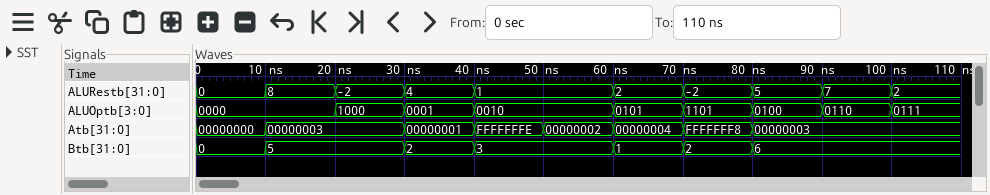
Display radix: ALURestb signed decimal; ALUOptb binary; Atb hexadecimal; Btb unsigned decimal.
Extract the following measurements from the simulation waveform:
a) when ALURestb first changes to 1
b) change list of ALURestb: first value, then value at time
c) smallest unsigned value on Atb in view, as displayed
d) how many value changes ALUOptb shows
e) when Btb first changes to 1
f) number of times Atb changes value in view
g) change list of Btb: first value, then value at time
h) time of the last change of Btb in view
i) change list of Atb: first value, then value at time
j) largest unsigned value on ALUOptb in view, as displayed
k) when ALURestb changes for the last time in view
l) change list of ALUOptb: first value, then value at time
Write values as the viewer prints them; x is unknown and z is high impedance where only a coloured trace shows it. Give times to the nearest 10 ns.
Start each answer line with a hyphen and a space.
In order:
- 40 ns
- 0, 8 at 10 ns, -2 at 20 ns, 4 at 30 ns, 1 at 40 ns, 2 at 60 ns, -2 at 70 ns, 5 at 80 ns, 7 at 90 ns, 2 at 100 ns
- 00000000
- 8
- 60 ns
- 7
- 0, 5 at 10 ns, 2 at 30 ns, 3 at 40 ns, 1 at 60 ns, 2 at 70 ns, 6 at 80 ns
- 80 ns
- 00000000, 00000003 at 10 ns, 00000001 at 30 ns, FFFFFFFE at 40 ns, 00000002 at 50 ns, 00000004 at 60 ns, FFFFFFF8 at 70 ns, 00000003 at 80 ns
- 1101
- 100 ns
- 0000, 1000 at 20 ns, 0001 at 30 ns, 0010 at 40 ns, 0101 at 60 ns, 1101 at 70 ns, 0100 at 80 ns, 0110 at 90 ns, 0111 at 100 ns
